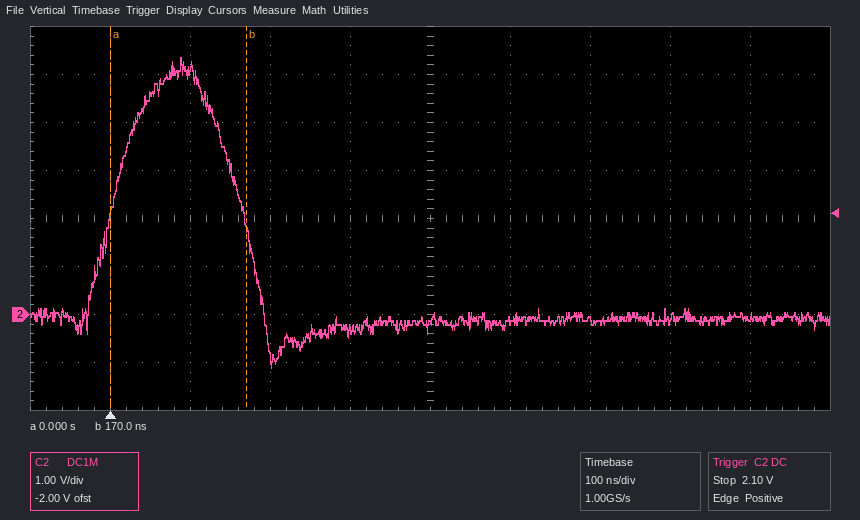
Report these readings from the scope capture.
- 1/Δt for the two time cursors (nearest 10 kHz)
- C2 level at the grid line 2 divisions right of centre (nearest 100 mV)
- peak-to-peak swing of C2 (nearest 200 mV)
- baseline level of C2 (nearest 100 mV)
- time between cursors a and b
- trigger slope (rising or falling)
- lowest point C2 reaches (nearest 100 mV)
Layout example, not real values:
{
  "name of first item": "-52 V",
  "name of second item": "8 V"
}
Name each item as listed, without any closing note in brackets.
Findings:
{
  "1/Δt for the two time cursors": "5.88 MHz",
  "C2 level at the grid line 2 divisions right of centre": "-100 mV",
  "peak-to-peak swing of C2": "6.4 V",
  "baseline level of C2": "-100 mV",
  "time between cursors a and b": "170 ns",
  "trigger slope": "rising",
  "lowest point C2 reaches": "-1.1 V"
}
